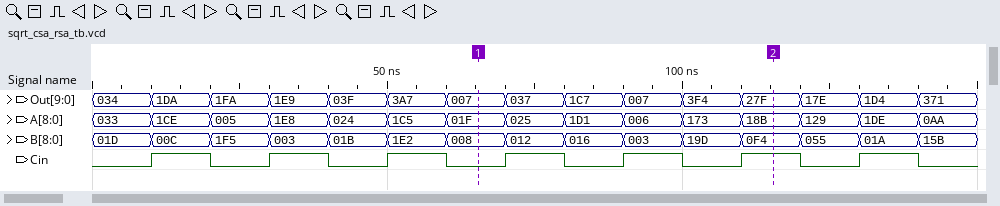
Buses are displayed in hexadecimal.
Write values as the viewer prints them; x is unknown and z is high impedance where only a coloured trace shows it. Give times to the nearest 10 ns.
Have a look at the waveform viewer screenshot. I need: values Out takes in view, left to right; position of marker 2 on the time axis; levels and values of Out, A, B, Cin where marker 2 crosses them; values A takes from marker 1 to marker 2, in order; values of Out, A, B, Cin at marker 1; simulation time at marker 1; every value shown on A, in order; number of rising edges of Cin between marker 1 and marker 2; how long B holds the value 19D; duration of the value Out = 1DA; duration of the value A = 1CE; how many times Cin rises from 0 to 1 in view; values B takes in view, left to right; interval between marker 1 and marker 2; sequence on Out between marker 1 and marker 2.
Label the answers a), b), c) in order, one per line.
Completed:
a) 034, 1DA, 1FA, 1E9, 03F, 3A7, 007, 037, 1C7, 007, 3F4, 27F, 17E, 1D4, 371
b) 120 ns
c) Out=27F, A=18B, B=0F4, Cin=1
d) 01F, 025, 1D1, 006, 173, 18B
e) Out=007, A=01F, B=008, Cin=0
f) 70 ns
g) 033, 1CE, 005, 1E8, 024, 1C5, 01F, 025, 1D1, 006, 173, 18B, 129, 1DE, 0AA
h) 3
i) 10 ns
j) 10 ns
k) 10 ns
l) 7
m) 01D, 00C, 1F5, 003, 01B, 1E2, 008, 012, 016, 003, 19D, 0F4, 055, 01A, 15B
n) 50 ns
o) 007, 037, 1C7, 007, 3F4, 27F
